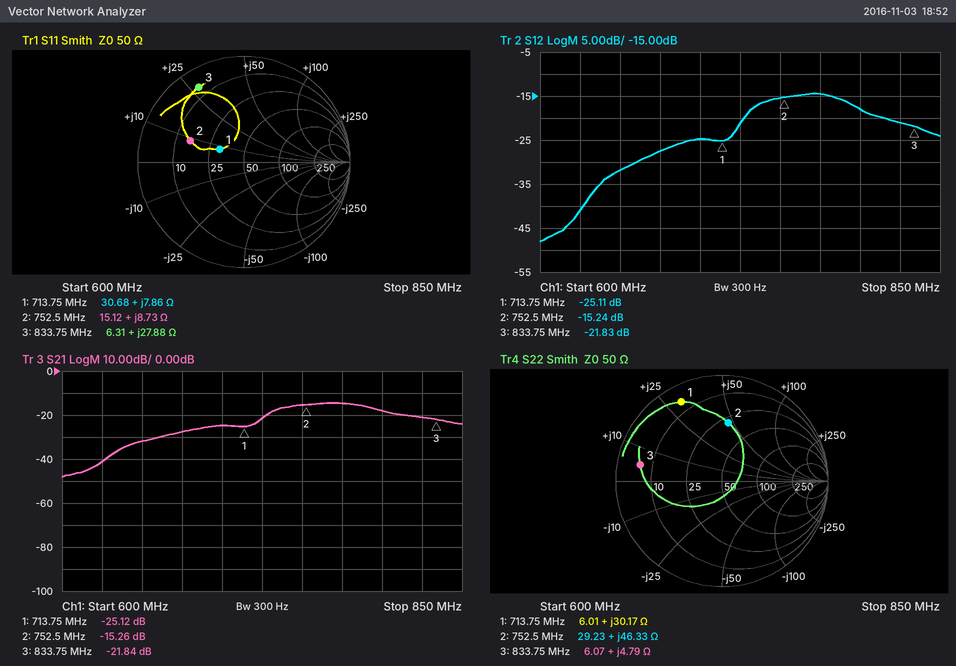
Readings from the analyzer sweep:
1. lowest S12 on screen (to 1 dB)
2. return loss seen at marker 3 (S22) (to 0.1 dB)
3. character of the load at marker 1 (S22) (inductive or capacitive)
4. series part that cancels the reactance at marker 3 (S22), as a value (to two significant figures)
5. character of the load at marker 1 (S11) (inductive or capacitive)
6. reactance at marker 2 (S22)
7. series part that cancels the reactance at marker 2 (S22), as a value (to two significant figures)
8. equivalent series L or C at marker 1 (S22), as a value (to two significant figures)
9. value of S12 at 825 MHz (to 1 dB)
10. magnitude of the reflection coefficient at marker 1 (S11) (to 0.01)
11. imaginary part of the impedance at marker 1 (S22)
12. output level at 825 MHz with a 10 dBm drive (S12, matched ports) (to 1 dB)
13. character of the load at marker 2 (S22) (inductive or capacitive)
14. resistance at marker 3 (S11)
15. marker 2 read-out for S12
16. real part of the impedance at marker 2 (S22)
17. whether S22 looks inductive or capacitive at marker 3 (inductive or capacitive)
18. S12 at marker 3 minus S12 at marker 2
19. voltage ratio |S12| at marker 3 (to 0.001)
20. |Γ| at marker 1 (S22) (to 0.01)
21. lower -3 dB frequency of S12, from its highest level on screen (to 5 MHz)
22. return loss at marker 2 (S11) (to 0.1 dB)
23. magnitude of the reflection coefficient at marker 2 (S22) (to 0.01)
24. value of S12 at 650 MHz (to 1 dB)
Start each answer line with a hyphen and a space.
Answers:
- -48 dB
- 2.1 dB
- inductive
- 40 pF
- inductive
- +46.33 Ω
- 4.6 pF
- 6.7 nH
- -21 dB
- 0.26
- +30.17 Ω
- -11 dBm
- inductive
- 6.31 Ω
- -15.24 dB
- 29.23 Ω
- inductive
- -6.59 dB
- 0.081
- 0.84
- 735 MHz
- 5.2 dB
- 0.55
- -32 dB
